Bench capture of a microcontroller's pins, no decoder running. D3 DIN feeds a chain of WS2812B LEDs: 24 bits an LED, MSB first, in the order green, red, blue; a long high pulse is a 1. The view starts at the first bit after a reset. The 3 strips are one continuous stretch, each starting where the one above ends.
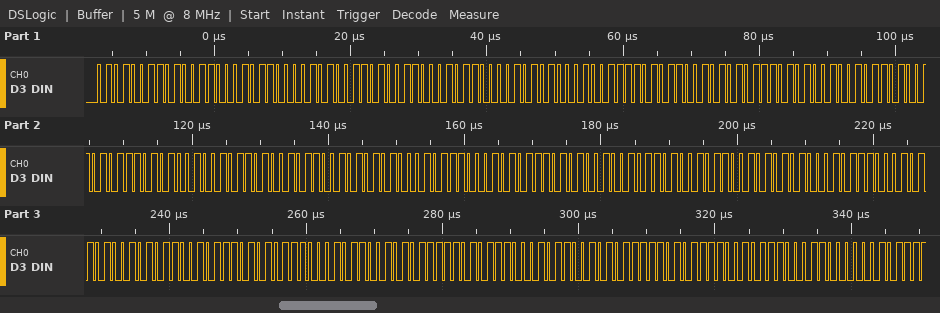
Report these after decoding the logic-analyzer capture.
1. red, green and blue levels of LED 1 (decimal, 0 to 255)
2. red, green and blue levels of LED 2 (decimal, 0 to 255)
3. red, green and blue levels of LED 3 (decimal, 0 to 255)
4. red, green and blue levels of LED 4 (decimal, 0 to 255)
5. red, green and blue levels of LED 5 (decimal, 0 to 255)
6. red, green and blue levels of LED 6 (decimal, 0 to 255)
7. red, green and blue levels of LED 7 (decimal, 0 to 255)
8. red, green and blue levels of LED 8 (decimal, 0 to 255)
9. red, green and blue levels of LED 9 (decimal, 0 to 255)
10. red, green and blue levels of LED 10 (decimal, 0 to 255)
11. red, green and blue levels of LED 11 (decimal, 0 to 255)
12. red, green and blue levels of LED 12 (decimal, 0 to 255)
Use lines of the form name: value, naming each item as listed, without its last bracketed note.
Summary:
red, green and blue levels of LED 1: 76, 83, 88
red, green and blue levels of LED 2: 76, 83, 88
red, green and blue levels of LED 3: 79, 84, 89
red, green and blue levels of LED 4: 82, 87, 90
red, green and blue levels of LED 5: 82, 87, 90
red, green and blue levels of LED 6: 84, 89, 92
red, green and blue levels of LED 7: 82, 87, 90
red, green and blue levels of LED 8: 84, 89, 92
red, green and blue levels of LED 9: 86, 90, 93
red, green and blue levels of LED 10: 89, 92, 95
red, green and blue levels of LED 11: 89, 92, 95
red, green and blue levels of LED 12: 92, 94, 96
